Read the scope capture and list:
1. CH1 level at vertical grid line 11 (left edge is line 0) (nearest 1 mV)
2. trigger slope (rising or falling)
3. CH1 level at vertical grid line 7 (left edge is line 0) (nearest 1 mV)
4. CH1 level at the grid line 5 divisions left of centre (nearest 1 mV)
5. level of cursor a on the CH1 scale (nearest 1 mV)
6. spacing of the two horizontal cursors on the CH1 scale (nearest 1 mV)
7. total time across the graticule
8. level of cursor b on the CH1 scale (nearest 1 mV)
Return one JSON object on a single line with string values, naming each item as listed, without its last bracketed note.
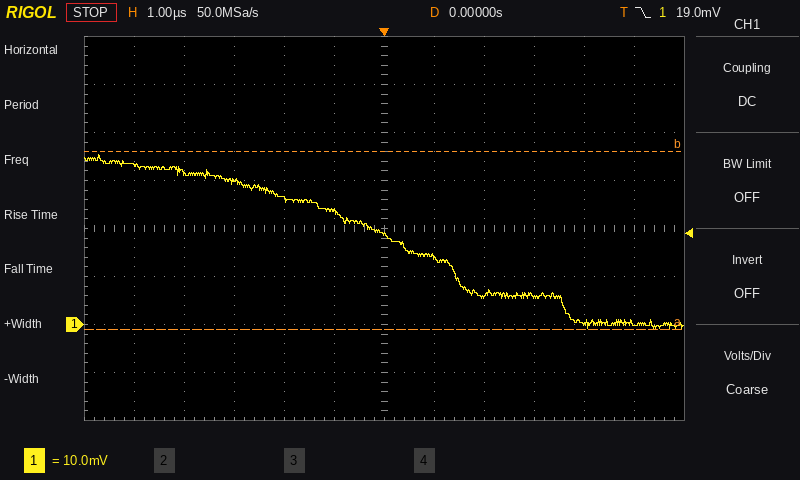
{"CH1 level at vertical grid line 11 (left edge is line 0)": "0 mV", "trigger slope": "falling", "CH1 level at vertical grid line 7 (left edge is line 0)": "14 mV", "CH1 level at the grid line 5 divisions left of centre": "33 mV", "level of cursor a on the CH1 scale": "-1 mV", "spacing of the two horizontal cursors on the CH1 scale": "37 mV", "total time across the graticule": "12 µs", "level of cursor b on the CH1 scale": "36 mV"}
